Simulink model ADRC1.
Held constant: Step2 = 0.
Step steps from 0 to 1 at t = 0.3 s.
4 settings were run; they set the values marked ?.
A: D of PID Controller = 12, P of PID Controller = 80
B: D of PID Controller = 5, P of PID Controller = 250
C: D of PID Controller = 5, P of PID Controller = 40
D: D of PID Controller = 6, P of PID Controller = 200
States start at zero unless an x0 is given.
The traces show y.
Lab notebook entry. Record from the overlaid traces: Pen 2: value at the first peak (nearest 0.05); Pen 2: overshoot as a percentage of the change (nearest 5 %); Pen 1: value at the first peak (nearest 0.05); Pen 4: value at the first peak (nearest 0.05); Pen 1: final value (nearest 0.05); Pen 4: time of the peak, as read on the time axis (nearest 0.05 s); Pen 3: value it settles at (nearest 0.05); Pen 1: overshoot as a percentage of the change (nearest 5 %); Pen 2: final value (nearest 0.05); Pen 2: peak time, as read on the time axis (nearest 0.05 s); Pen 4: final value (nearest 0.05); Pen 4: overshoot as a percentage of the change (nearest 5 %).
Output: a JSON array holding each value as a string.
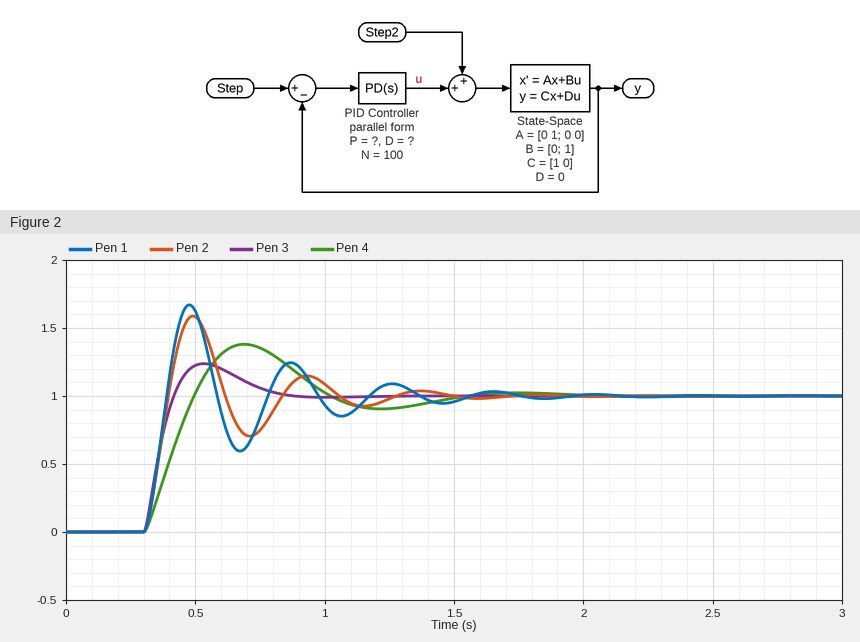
["1.60", "60 %", "1.65", "1.40", "1.00", "0.70 s", "1.00", "65 %", "1.00", "0.50 s", "1.00", "40 %"]
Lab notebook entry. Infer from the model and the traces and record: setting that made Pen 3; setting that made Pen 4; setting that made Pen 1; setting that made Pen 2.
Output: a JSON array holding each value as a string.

["A", "C", "B", "D"]
